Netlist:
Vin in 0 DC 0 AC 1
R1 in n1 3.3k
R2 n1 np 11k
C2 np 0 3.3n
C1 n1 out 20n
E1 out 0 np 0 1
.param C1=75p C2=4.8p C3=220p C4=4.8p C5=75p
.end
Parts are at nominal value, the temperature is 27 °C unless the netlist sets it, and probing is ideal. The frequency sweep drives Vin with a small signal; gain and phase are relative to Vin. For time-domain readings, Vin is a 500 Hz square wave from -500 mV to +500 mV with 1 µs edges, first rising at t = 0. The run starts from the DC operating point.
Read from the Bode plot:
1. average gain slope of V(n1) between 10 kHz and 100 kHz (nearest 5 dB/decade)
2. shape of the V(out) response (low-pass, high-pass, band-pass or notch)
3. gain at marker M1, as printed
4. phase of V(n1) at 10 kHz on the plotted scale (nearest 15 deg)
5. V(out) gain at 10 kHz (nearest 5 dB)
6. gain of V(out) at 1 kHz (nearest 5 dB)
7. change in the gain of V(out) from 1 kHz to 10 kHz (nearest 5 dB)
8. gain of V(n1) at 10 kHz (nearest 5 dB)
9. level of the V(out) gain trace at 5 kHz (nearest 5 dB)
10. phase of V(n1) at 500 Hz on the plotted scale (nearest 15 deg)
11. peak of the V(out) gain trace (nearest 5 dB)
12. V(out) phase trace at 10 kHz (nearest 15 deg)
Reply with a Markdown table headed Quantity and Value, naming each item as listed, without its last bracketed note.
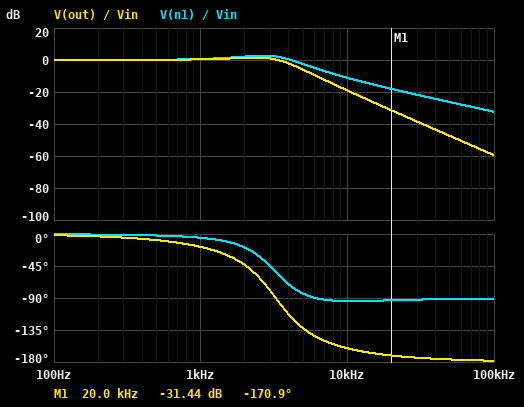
| Quantity | Value |
|---|---|
| average gain slope of V(n1) between 10 kHz and 100 kHz | -20 dB/decade |
| shape of the V(out) response | low-pass |
| gain at marker M1, as printed | -31.44 dB |
| phase of V(n1) at 10 kHz on the plotted scale | -90 deg |
| V(out) gain at 10 kHz | -20 dB |
| gain of V(out) at 1 kHz | 0 dB |
| change in the gain of V(out) from 1 kHz to 10 kHz | -20 dB |
| gain of V(n1) at 10 kHz | -10 dB |
| level of the V(out) gain trace at 5 kHz | -5 dB |
| phase of V(n1) at 500 Hz on the plotted scale | 0 deg |
| peak of the V(out) gain trace | 0 dB |
| V(out) phase trace at 10 kHz | -165 deg |
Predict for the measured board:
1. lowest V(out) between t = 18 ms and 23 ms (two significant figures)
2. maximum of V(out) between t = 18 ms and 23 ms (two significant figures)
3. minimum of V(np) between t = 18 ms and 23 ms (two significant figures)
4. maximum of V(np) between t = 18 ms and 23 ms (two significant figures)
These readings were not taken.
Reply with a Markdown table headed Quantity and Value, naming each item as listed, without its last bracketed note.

| Quantity | Value |
|---|---|
| lowest V(out) between t = 18 ms and 23 ms | -680 mV |
| maximum of V(out) between t = 18 ms and 23 ms | 680 mV |
| minimum of V(np) between t = 18 ms and 23 ms | -680 mV |
| maximum of V(np) between t = 18 ms and 23 ms | 680 mV |
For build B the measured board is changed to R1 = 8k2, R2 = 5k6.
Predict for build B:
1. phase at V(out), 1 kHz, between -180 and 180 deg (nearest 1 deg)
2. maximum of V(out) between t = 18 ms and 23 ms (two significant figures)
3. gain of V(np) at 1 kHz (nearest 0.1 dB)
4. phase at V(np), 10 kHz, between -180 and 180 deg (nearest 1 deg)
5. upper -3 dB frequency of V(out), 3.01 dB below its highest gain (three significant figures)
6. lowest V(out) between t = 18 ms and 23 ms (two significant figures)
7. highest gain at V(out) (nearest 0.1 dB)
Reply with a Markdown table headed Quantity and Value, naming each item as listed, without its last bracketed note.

| Quantity | Value |
|---|---|
| phase at V(out), 1 kHz, between -180 and 180 deg | -18 deg |
| maximum of V(out) between t = 18 ms and 23 ms | 740 mV |
| gain of V(np) at 1 kHz | 0.7 dB |
| phase at V(np), 10 kHz, between -180 and 180 deg | -165 deg |
| upper -3 dB frequency of V(out), 3.01 dB below its highest gain | 3.43 kHz |
| lowest V(out) between t = 18 ms and 23 ms | -740 mV |
| highest gain at V(out) | 2.5 dB |
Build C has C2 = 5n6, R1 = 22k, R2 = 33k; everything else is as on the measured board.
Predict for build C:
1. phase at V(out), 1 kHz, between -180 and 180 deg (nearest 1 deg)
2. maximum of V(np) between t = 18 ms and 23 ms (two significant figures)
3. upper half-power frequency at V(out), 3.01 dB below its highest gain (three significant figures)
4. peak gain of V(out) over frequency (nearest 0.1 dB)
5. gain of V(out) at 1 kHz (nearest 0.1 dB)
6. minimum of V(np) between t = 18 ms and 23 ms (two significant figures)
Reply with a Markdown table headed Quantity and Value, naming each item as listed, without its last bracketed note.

| Quantity | Value |
|---|---|
| phase at V(out), 1 kHz, between -180 and 180 deg | -139 deg |
| maximum of V(np) between t = 18 ms and 23 ms | 650 mV |
| upper half-power frequency at V(out), 3.01 dB below its highest gain | 643 Hz |
| peak gain of V(out) over frequency | 0.8 dB |
| gain of V(out) at 1 kHz | -9.4 dB |
| minimum of V(np) between t = 18 ms and 23 ms | -650 mV |
